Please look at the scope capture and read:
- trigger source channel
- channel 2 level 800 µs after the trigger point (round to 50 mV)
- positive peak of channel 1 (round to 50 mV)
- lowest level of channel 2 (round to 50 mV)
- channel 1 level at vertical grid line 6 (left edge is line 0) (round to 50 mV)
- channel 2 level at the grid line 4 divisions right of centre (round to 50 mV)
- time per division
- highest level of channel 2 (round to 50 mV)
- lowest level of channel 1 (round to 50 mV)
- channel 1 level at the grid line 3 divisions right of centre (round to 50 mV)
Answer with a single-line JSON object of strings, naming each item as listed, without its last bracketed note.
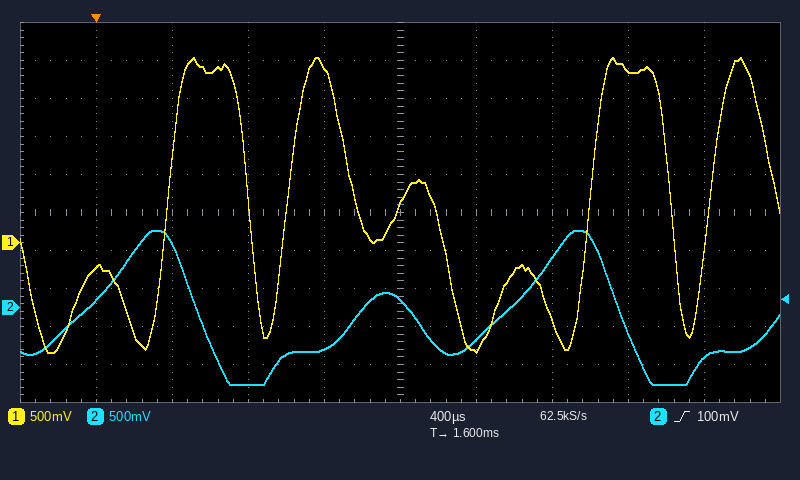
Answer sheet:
{"trigger source channel": "channel 2", "channel 2 level 800 µs after the trigger point": "-1.00 V", "positive peak of channel 1": "2.45 V", "lowest level of channel 2": "-1.00 V", "channel 1 level at vertical grid line 6 (left edge is line 0)": "-1.40 V", "channel 2 level at the grid line 4 divisions right of centre": "-650 mV", "time per division": "400 µs", "highest level of channel 2": "1.00 V", "lowest level of channel 1": "-1.45 V", "channel 1 level at the grid line 3 divisions right of centre": "2.30 V"}
